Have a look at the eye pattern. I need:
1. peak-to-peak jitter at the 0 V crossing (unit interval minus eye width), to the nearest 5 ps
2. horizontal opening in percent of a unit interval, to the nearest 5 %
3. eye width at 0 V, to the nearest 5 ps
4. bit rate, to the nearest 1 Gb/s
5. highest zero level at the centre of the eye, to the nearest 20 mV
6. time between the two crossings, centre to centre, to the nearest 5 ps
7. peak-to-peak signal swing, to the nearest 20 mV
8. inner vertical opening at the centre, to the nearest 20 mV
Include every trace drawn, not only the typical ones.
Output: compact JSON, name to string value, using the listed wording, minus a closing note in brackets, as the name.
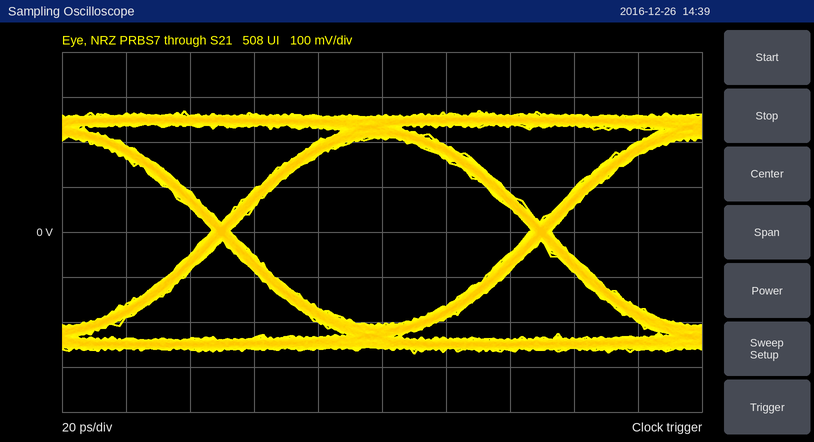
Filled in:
{"peak-to-peak jitter at the 0 V crossing (unit interval minus eye width), to the nearest 5 ps": "5 ps", "horizontal opening in percent of a unit interval, to the nearest 5 %": "95 %", "eye width at 0 V, to the nearest 5 ps": "95 ps", "bit rate, to the nearest 1 Gb/s": "10 Gb/s", "highest zero level at the centre of the eye, to the nearest 20 mV": "-200 mV", "time between the two crossings, centre to centre, to the nearest 5 ps": "100 ps", "peak-to-peak signal swing, to the nearest 20 mV": "540 mV", "inner vertical opening at the centre, to the nearest 20 mV": "420 mV"}
